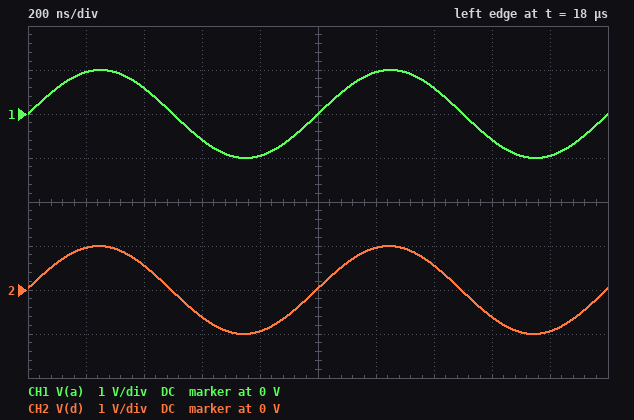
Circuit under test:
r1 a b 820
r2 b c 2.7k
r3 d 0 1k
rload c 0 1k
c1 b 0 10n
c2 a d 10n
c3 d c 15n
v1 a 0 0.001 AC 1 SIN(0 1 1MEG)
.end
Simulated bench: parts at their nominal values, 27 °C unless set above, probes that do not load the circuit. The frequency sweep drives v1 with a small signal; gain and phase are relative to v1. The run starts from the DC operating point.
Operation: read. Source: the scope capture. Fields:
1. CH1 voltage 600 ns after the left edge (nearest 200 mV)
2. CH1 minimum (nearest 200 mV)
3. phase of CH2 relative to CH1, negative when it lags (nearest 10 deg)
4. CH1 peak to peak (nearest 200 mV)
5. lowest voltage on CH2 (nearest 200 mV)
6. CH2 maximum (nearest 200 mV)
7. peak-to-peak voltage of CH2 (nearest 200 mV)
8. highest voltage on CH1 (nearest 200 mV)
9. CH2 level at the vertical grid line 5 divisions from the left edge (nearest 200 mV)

-600 mV
-1.0 V
0 deg
2.0 V
-1.0 V
1.0 V
2.0 V
1.0 V
0 V
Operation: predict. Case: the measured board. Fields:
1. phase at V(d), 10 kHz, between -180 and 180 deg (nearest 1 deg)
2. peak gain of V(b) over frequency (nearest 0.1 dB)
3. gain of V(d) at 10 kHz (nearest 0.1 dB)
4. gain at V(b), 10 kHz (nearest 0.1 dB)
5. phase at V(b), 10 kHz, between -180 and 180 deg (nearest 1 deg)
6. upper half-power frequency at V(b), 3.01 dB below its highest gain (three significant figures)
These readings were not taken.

39 deg
-1.7 dB
-8.4 dB
-2.7 dB
-20 deg
24.7 kHz
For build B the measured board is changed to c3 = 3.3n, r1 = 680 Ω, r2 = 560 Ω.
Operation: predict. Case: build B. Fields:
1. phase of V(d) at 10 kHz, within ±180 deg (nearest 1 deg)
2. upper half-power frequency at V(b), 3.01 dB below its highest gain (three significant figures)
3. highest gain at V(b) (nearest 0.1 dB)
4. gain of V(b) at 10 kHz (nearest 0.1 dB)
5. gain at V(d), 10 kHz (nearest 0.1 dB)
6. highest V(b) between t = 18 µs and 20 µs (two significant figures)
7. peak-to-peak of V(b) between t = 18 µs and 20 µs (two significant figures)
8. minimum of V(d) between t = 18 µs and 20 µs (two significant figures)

48 deg
28.1 kHz
-3.1 dB
-3.9 dB
-5.4 dB
52 mV
100 mV
-990 mV
